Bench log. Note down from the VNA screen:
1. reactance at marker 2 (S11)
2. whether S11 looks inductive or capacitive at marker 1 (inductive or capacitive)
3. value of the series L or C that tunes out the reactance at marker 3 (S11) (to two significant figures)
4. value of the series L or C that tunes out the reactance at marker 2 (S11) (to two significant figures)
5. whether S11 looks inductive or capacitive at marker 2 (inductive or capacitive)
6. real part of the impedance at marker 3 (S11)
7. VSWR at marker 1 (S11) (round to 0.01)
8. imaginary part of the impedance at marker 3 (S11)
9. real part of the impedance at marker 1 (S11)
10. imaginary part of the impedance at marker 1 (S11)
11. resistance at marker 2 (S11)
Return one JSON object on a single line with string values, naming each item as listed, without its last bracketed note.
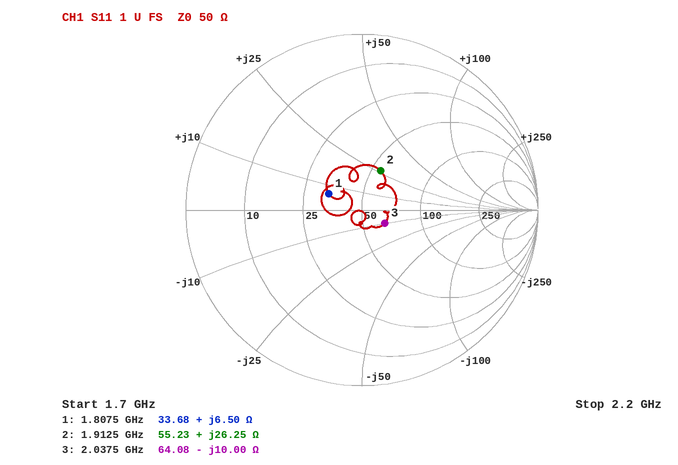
{"reactance at marker 2": "+26.25 Ω", "whether S11 looks inductive or capacitive at marker 1": "inductive", "value of the series L or C that tunes out the reactance at marker 3 (S11)": "780 pH", "value of the series L or C that tunes out the reactance at marker 2 (S11)": "3.2 pF", "whether S11 looks inductive or capacitive at marker 2": "inductive", "real part of the impedance at marker 3": "64.08 Ω", "VSWR at marker 1 (S11)": "1.53", "imaginary part of the impedance at marker 3": "-10.00 Ω", "real part of the impedance at marker 1": "33.68 Ω", "imaginary part of the impedance at marker 1": "+6.50 Ω", "resistance at marker 2": "55.23 Ω"}
